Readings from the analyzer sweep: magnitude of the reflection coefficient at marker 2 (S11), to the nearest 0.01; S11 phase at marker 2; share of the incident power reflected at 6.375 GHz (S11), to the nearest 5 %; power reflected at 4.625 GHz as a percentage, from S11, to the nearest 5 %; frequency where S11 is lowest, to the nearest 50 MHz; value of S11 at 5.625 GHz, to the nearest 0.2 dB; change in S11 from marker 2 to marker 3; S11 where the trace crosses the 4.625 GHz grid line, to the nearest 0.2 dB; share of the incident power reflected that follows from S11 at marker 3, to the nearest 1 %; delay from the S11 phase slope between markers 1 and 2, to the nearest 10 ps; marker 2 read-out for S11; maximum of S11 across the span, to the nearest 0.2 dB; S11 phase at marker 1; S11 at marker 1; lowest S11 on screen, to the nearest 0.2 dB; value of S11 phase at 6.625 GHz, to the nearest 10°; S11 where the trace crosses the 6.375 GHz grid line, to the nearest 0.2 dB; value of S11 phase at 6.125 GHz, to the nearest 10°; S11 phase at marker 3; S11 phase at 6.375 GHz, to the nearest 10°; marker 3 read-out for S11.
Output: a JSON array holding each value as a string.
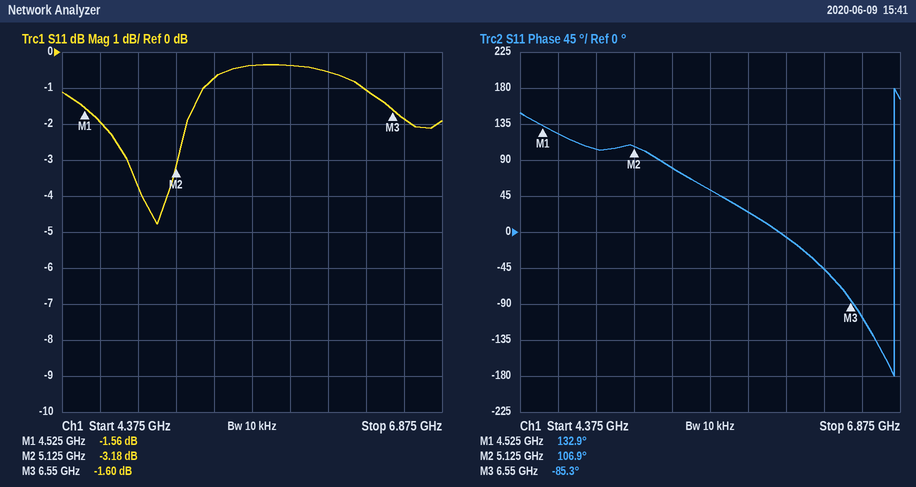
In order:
["0.69", "106.9°", "80 %", "65 %", "5.00 GHz", "-0.4 dB", "1.58 dB", "-2.0 dB", "69 %", "120 ps", "-3.18 dB", "-0.4 dB", "132.9°", "-1.56 dB", "-4.8 dB", "-110°", "-1.0 dB", "-10°", "-85.3°", "-50°", "-1.60 dB"]
